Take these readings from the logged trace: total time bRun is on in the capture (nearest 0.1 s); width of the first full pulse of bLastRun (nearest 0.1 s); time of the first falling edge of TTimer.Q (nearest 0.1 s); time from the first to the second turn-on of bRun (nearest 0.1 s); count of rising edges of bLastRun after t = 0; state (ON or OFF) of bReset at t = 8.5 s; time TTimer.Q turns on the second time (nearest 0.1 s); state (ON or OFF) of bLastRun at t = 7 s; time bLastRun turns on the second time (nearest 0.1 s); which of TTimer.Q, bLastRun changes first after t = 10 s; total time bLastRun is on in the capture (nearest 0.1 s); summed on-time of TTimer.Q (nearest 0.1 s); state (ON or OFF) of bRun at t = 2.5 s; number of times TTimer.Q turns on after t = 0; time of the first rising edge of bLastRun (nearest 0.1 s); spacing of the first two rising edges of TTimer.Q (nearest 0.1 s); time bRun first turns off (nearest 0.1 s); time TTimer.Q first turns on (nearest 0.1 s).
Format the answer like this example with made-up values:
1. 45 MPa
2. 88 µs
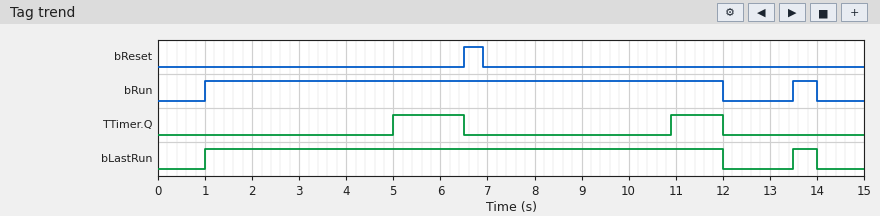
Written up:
1. 11.5 s
2. 11.0 s
3. 6.5 s
4. 12.5 s
5. 2
6. OFF
7. 10.9 s
8. ON
9. 13.5 s
10. TTimer.Q
11. 11.5 s
12. 2.6 s
13. ON
14. 2
15. 1.0 s
16. 5.9 s
17. 12.0 s
18. 5.0 s
